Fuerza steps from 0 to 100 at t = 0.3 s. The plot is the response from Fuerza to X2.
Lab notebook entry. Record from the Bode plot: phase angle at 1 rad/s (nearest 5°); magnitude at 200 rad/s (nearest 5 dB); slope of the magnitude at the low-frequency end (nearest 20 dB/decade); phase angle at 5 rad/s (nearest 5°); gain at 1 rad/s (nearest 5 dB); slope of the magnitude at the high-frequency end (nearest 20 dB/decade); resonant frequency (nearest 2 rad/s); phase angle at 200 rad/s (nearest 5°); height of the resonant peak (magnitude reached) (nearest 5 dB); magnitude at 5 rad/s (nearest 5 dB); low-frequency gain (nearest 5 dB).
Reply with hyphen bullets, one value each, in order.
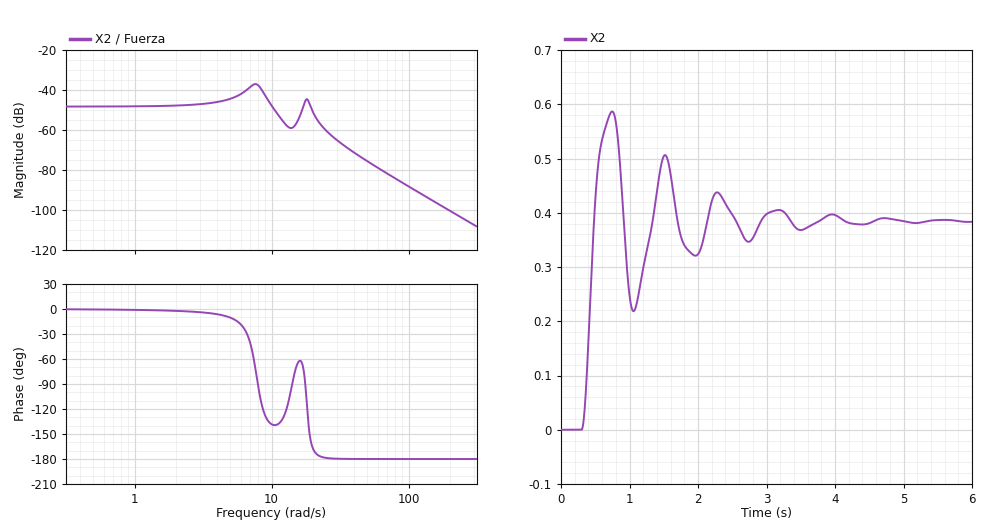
- 0°
- -100 dB
- 0 dB/decade
- -10°
- -50 dB
- -40 dB/decade
- 8 rad/s
- -180°
- -35 dB
- -45 dB
- -50 dB
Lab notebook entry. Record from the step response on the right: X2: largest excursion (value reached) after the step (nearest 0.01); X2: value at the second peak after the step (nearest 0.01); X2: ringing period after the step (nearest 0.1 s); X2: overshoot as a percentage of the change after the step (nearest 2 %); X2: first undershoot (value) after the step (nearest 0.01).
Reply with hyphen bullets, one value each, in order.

- 0.59
- 0.51
- 0.8 s
- 52 %
- 0.22
